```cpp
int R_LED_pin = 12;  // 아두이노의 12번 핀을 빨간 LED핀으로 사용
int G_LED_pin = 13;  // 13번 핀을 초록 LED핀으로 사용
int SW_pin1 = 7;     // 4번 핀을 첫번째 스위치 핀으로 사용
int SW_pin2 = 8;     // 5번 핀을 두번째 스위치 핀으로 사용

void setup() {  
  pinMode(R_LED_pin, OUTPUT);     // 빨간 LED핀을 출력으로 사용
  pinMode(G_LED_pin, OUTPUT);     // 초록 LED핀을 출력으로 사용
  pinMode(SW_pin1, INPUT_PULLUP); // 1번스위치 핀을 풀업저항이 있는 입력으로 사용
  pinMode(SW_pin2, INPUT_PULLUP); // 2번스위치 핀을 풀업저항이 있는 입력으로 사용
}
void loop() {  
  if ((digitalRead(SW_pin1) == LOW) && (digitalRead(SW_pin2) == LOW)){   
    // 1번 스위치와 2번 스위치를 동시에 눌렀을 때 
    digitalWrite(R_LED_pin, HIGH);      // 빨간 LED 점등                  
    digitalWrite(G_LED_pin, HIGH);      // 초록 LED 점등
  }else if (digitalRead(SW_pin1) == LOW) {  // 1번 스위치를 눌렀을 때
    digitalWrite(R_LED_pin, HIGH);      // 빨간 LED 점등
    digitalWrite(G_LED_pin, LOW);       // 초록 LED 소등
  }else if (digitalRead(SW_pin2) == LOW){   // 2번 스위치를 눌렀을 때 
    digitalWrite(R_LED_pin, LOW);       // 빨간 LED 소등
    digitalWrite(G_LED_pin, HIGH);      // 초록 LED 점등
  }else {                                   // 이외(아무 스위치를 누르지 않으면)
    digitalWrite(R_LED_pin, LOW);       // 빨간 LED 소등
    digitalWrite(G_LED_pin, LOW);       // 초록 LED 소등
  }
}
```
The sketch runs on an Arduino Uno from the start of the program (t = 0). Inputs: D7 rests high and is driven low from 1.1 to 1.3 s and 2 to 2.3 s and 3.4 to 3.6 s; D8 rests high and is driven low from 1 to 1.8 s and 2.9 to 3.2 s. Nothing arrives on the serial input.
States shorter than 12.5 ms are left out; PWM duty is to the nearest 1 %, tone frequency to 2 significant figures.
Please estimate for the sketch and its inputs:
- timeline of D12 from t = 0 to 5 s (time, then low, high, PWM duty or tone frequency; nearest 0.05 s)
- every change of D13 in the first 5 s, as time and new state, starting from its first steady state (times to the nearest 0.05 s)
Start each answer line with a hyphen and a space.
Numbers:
- 0 s low; 1.1 s high; 1.3 s low; 2 s high; 2.3 s low; 3.4 s high; 3.6 s low
- 0 s low; 1 s high; 1.8 s low; 2.9 s high; 3.2 s low
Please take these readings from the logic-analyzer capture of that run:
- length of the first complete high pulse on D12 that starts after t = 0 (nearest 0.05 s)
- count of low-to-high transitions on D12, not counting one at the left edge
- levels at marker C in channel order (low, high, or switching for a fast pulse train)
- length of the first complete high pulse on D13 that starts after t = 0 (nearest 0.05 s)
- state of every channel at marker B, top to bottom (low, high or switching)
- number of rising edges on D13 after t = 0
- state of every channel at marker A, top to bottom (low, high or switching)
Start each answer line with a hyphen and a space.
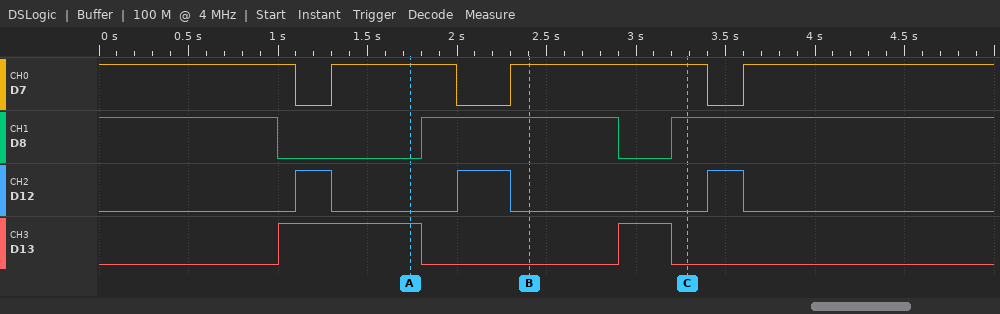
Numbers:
- 0.20 s
- 3
- D7 high, D8 high, D12 low, D13 low
- 0.80 s
- D7 high, D8 high, D12 low, D13 low
- 2
- D7 high, D8 low, D12 low, D13 high
